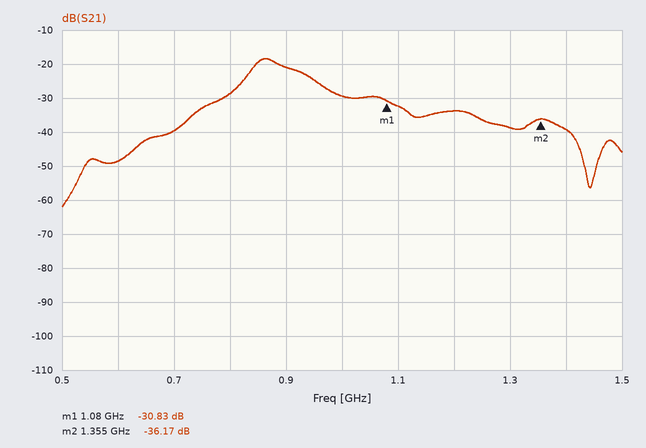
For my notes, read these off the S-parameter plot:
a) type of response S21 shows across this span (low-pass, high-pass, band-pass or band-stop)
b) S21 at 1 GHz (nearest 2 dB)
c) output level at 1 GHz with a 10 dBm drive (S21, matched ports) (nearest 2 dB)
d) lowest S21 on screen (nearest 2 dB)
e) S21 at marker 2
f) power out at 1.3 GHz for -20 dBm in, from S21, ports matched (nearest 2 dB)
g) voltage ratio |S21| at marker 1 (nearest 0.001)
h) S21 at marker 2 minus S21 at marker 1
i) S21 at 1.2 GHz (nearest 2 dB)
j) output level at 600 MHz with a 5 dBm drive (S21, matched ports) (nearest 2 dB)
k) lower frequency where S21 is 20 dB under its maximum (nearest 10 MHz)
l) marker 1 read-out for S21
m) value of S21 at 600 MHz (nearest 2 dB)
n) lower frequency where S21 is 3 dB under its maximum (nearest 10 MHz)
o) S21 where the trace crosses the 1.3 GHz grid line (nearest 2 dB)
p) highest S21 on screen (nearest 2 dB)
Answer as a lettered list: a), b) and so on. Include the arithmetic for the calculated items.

a) band-pass
b) -30 dB
c) 10 dBm + (-30 dB) = -20 dBm
d) -62 dB
e) -36.17 dB
f) -20 dBm + (-38 dB) = -58 dBm
g) 10^(-30.83/20) ≈ 0.029
h) -36.17 − (-30.83) = -5.34 dB
i) -34 dB
j) 5 dBm + (-48 dB) = -44 dBm
k) 710 MHz
l) -30.83 dB
m) -48 dB
n) 840 MHz
o) -38 dB
p) -18 dB
